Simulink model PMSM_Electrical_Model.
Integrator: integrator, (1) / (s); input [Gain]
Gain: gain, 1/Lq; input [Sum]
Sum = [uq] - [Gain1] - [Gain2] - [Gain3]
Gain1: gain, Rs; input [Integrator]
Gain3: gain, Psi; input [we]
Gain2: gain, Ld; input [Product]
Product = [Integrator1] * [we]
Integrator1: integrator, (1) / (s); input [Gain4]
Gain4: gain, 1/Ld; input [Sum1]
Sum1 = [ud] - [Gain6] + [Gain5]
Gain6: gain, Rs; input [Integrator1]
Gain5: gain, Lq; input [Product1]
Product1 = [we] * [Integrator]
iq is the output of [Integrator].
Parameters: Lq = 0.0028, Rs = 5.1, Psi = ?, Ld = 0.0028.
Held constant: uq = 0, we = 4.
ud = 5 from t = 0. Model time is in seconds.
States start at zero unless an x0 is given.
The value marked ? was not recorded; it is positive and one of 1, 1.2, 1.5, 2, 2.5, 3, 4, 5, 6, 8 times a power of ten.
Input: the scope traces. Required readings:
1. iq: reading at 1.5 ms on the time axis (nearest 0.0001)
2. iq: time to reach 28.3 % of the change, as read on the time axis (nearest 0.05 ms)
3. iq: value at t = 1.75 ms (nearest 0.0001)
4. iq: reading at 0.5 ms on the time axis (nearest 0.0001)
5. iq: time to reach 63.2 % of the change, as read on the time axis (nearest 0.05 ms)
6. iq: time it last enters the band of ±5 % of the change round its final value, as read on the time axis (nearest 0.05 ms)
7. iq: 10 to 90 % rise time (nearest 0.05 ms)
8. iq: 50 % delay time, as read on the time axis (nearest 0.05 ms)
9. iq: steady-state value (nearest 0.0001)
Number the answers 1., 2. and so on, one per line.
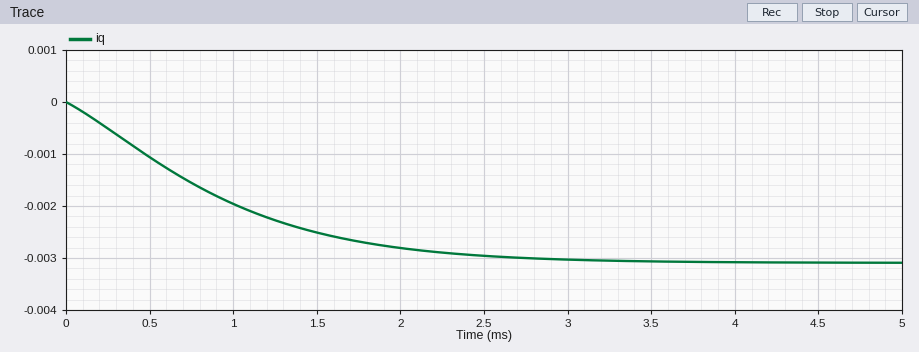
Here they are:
1. -0.0025
2. 0.40 ms
3. -0.0027
4. -0.0011
5. 1.00 ms
6. 2.40 ms
7. 1.80 ms
8. 0.75 ms
9. -0.0031
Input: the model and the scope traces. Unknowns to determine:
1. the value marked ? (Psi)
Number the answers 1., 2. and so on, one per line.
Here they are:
1. 0.0012
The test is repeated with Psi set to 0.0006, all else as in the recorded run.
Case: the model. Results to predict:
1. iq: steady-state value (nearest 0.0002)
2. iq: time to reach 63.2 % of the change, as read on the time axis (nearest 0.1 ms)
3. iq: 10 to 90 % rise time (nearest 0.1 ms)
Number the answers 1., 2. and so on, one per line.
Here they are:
1. -0.0026
2. 1.1 ms
3. 1.8 ms
